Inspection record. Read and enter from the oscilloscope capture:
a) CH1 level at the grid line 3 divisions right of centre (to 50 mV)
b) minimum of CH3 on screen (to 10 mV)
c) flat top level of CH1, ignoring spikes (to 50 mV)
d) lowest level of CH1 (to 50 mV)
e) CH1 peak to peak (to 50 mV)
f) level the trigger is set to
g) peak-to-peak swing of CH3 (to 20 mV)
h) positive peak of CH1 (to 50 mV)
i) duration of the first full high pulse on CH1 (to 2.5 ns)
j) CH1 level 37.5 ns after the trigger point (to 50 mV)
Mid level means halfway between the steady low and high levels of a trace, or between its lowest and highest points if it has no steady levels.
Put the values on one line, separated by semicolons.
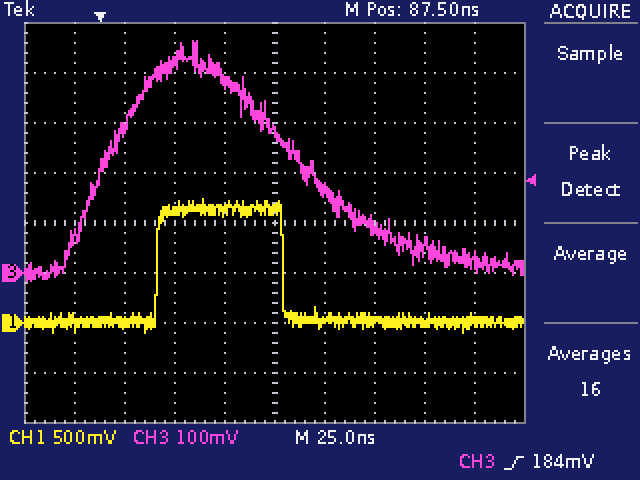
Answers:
0 mV; -20 mV; 1.15 V; -100 mV; 1.35 V; 184 mV; 480 mV; 1.25 V; 62.5 ns; 1.10 V
